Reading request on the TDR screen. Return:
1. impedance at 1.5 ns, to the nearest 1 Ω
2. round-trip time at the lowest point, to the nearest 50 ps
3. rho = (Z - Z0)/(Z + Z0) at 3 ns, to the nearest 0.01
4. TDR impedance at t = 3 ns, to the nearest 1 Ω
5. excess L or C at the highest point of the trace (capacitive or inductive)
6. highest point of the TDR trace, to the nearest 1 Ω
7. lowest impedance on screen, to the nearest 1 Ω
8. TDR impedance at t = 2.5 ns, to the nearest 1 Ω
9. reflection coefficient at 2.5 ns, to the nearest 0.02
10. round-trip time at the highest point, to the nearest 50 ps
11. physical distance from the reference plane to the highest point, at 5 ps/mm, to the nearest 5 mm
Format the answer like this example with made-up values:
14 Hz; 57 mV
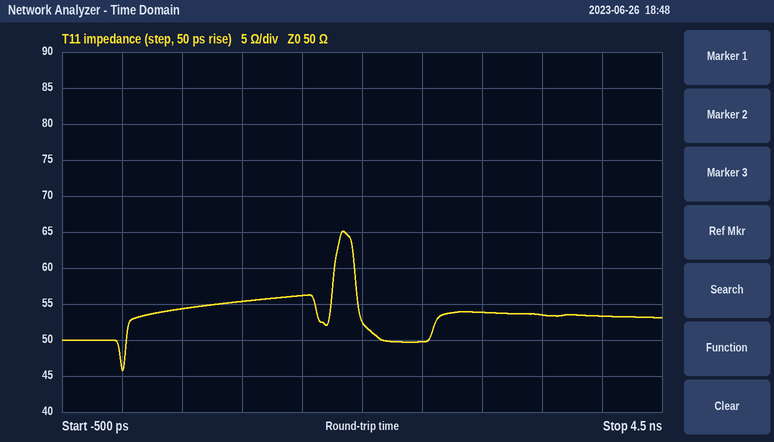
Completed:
56 Ω; 0 ps; +0.04; 54 Ω; inductive; 65 Ω; 46 Ω; 50 Ω; 0.00; 1.85 ns; 185 mm
